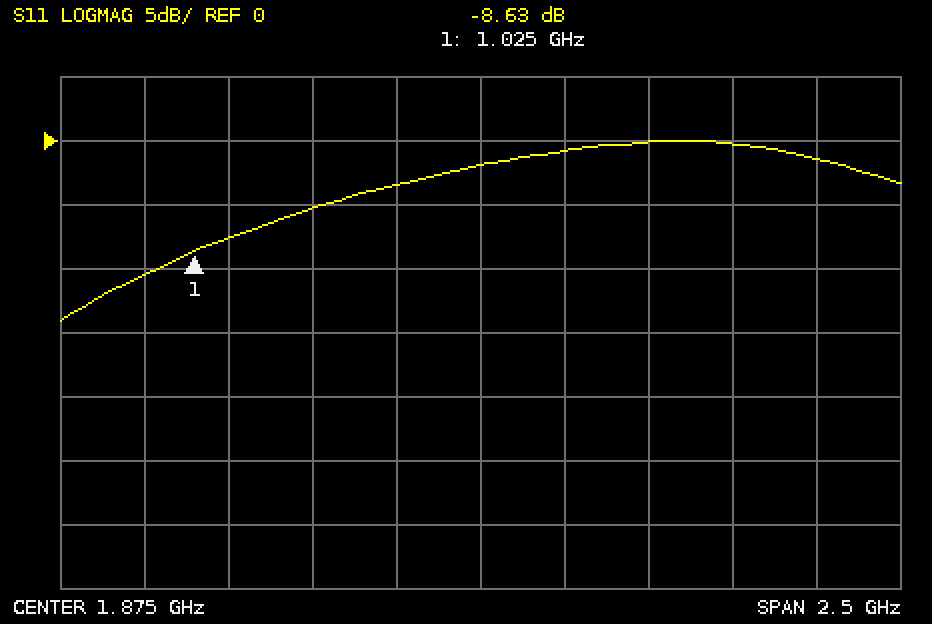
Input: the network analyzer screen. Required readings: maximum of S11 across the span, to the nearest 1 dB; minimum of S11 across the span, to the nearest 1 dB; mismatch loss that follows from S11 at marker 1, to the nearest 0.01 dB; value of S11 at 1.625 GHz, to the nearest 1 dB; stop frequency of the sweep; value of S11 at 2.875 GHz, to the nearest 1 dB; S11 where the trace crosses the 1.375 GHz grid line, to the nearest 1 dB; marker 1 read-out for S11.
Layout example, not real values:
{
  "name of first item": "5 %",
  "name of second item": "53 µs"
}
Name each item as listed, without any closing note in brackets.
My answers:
{
  "maximum of S11 across the span, to the nearest 1 dB": "0 dB",
  "minimum of S11 across the span, to the nearest 1 dB": "-14 dB",
  "mismatch loss that follows from S11 at marker 1, to the nearest 0.01 dB": "0.64 dB",
  "value of S11 at 1.625 GHz, to the nearest 1 dB": "-3 dB",
  "stop frequency of the sweep": "3.125 GHz",
  "value of S11 at 2.875 GHz, to the nearest 1 dB": "-1 dB",
  "S11 where the trace crosses the 1.375 GHz grid line, to the nearest 1 dB": "-5 dB",
  "marker 1 read-out for S11": "-8.63 dB"
}
